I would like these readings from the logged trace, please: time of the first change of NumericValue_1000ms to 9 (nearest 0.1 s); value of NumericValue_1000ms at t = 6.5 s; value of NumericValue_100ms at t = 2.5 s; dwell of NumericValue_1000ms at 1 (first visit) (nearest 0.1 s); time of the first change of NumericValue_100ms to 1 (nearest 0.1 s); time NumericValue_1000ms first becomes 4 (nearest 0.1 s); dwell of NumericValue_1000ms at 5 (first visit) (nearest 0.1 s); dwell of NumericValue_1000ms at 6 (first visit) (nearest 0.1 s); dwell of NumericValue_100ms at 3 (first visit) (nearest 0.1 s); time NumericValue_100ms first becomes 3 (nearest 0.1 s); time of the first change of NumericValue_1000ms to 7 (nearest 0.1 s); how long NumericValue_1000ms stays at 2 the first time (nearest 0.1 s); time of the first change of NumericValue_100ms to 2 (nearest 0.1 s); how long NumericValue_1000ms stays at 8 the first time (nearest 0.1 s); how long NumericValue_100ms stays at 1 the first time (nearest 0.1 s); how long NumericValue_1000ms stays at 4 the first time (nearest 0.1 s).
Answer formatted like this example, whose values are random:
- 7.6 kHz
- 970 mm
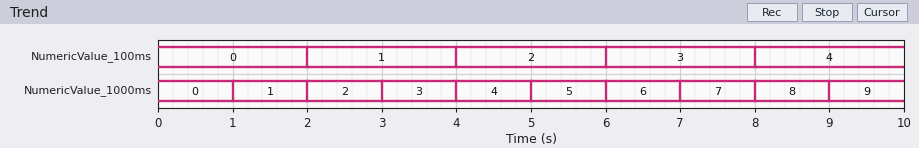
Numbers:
- 9.0 s
- 6
- 1
- 1.0 s
- 2.0 s
- 4.0 s
- 1.0 s
- 1.0 s
- 2.0 s
- 6.0 s
- 7.0 s
- 1.0 s
- 4.0 s
- 1.0 s
- 2.0 s
- 1.0 s
